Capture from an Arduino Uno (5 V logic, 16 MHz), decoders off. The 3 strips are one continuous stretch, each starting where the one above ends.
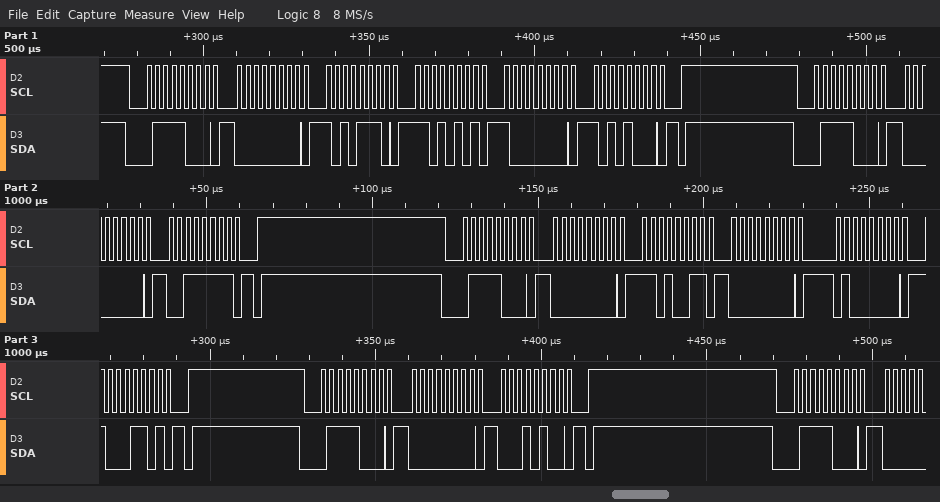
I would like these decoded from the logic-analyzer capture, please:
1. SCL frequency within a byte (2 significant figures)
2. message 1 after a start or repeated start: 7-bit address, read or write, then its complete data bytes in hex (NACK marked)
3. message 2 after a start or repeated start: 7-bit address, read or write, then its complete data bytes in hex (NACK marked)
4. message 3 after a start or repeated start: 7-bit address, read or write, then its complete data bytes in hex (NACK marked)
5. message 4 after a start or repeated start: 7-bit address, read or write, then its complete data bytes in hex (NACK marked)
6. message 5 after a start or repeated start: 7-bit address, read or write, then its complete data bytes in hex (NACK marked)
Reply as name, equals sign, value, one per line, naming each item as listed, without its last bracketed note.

SCL frequency within a byte = 400 kHz
message 1 after a start or repeated start: 7-bit address, read or write, then its complete data bytes in hex = 0x3C write: 00 AE D5 80 A8
message 2 after a start or repeated start: 7-bit address, read or write, then its complete data bytes in hex = 0x3C write: 00 3F
message 3 after a start or repeated start: 7-bit address, read or write, then its complete data bytes in hex = 0x3C write: 00 D3 00 40 8D
message 4 after a start or repeated start: 7-bit address, read or write, then its complete data bytes in hex = 0x3C write: 00 14
message 5 after a start or repeated start: 7-bit address, read or write, then its complete data bytes in hex = 0x3C write
